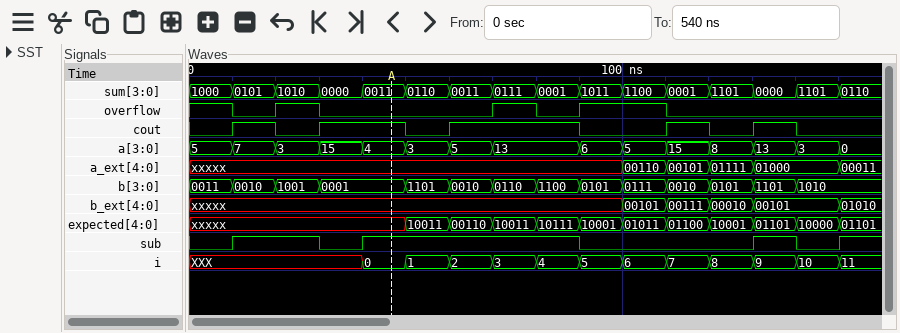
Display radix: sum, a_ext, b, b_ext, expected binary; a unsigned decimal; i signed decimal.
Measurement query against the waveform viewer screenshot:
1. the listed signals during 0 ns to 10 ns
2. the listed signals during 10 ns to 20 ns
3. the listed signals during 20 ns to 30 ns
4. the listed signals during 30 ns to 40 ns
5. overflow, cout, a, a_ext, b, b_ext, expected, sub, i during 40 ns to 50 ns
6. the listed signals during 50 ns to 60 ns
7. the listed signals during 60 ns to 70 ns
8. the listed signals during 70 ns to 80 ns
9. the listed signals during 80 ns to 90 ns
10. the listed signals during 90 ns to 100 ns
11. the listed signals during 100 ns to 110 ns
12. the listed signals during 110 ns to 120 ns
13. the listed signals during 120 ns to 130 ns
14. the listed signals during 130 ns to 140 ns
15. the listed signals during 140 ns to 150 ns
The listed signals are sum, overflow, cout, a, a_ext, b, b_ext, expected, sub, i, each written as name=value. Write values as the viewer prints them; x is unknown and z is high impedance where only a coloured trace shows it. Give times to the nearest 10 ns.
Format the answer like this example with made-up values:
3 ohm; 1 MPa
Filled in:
sum=1000, overflow=1, cout=0, a=5, a_ext=xxxxx, b=0011, b_ext=xxxxx, expected=xxxxx, sub=0, i=XXX; sum=0101, overflow=0, cout=1, a=7, a_ext=xxxxx, b=0010, b_ext=xxxxx, expected=xxxxx, sub=1, i=XXX; sum=1010, overflow=1, cout=0, a=3, a_ext=xxxxx, b=1001, b_ext=xxxxx, expected=xxxxx, sub=1, i=XXX; sum=0000, overflow=0, cout=1, a=15, a_ext=xxxxx, b=0001, b_ext=xxxxx, expected=xxxxx, sub=0, i=XXX; overflow=0, cout=1, a=4, a_ext=xxxxx, b=0001, b_ext=xxxxx, expected=xxxxx, sub=1, i=0; sum=0110, overflow=0, cout=0, a=3, a_ext=xxxxx, b=1101, b_ext=xxxxx, expected=10011, sub=1, i=1; sum=0011, overflow=0, cout=1, a=5, a_ext=xxxxx, b=0010, b_ext=xxxxx, expected=00110, sub=1, i=2; sum=0111, overflow=1, cout=1, a=13, a_ext=xxxxx, b=0110, b_ext=xxxxx, expected=10011, sub=1, i=3; sum=0001, overflow=0, cout=1, a=13, a_ext=xxxxx, b=1100, b_ext=xxxxx, expected=10111, sub=1, i=4; sum=1011, overflow=1, cout=0, a=6, a_ext=xxxxx, b=0101, b_ext=xxxxx, expected=10001, sub=0, i=5; sum=1100, overflow=1, cout=0, a=5, a_ext=00110, b=0111, b_ext=00101, expected=01011, sub=0, i=6; sum=0001, overflow=0, cout=1, a=15, a_ext=00101, b=0010, b_ext=00111, expected=01100, sub=0, i=7; sum=1101, overflow=0, cout=0, a=8, a_ext=01111, b=0101, b_ext=00010, expected=10001, sub=0, i=8; sum=0000, overflow=0, cout=1, a=13, a_ext=01000, b=1101, b_ext=00101, expected=01101, sub=1, i=9; sum=1101, overflow=0, cout=0, a=3, a_ext=01000, b=1010, b_ext=00101, expected=10000, sub=0, i=10
